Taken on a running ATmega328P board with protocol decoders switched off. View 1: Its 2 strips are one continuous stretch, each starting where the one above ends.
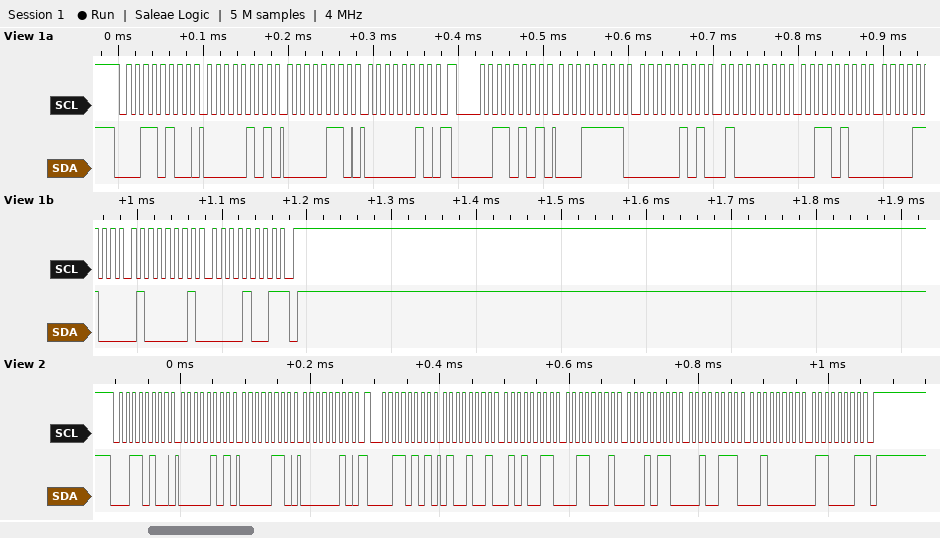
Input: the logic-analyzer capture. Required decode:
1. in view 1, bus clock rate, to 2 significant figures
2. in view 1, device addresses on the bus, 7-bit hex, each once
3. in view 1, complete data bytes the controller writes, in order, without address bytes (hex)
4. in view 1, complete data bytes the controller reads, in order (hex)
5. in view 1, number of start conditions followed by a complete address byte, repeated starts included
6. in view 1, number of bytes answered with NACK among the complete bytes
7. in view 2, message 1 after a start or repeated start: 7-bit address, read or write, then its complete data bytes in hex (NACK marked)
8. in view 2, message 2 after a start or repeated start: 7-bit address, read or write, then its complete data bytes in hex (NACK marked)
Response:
100 kHz
0x1A
05 06 02
1F 05 40 34 0C 41 09
2
1
0x1A write: 05 06 02
0x1A read: 49 53 31 16 27 20 61 NACK
